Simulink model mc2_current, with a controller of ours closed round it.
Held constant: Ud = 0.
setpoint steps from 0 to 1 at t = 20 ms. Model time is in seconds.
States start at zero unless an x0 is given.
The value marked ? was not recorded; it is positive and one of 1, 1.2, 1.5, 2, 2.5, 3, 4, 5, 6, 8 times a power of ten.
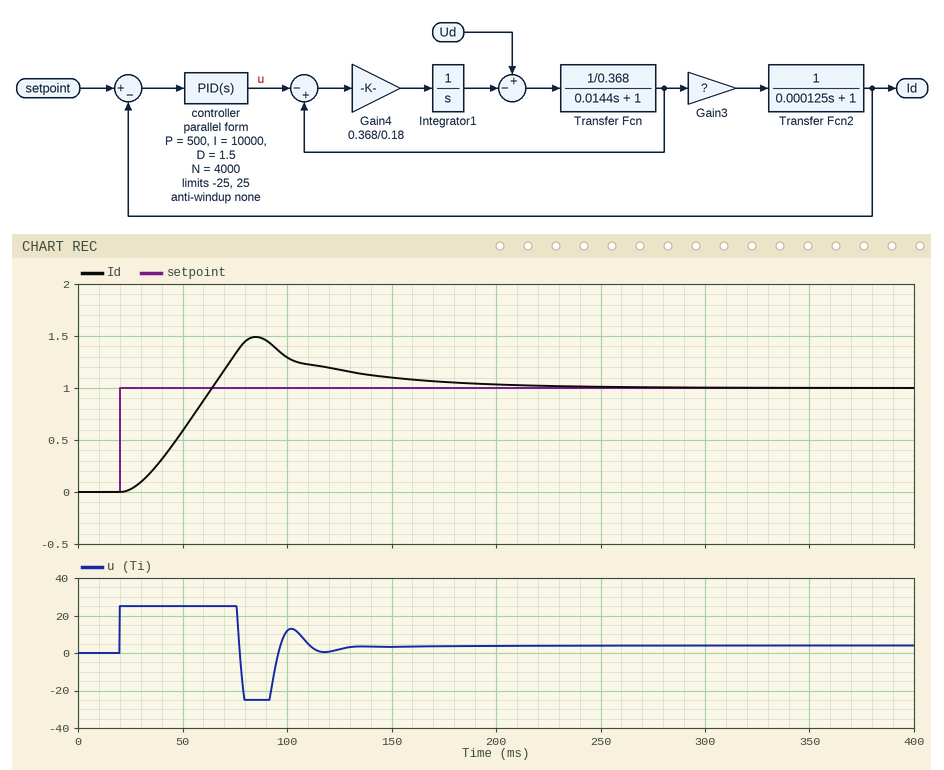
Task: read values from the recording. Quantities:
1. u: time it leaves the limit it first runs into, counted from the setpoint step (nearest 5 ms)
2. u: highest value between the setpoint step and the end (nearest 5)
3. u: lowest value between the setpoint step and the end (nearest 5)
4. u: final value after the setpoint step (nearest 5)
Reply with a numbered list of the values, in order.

1. 55 ms
2. 25
3. -25
4. 5
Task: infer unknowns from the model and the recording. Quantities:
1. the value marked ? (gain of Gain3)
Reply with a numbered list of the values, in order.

1. 0.25
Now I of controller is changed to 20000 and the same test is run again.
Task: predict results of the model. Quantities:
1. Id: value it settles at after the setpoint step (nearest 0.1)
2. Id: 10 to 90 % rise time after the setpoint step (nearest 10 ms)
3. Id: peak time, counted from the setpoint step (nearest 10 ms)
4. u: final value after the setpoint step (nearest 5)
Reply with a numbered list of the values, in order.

1. 1.0
2. 30 ms
3. 70 ms
4. 5
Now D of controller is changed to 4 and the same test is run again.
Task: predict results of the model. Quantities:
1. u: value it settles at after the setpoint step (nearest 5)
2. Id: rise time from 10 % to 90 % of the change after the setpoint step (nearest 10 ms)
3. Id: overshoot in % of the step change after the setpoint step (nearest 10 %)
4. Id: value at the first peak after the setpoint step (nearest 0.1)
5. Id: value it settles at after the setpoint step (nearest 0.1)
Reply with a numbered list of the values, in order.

1. 5
2. 30 ms
3. 40 %
4. 1.4
5. 1.0
